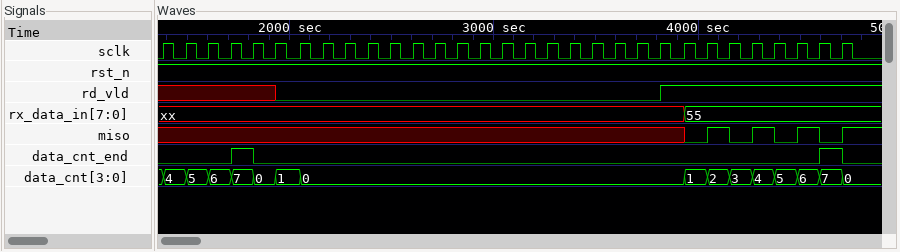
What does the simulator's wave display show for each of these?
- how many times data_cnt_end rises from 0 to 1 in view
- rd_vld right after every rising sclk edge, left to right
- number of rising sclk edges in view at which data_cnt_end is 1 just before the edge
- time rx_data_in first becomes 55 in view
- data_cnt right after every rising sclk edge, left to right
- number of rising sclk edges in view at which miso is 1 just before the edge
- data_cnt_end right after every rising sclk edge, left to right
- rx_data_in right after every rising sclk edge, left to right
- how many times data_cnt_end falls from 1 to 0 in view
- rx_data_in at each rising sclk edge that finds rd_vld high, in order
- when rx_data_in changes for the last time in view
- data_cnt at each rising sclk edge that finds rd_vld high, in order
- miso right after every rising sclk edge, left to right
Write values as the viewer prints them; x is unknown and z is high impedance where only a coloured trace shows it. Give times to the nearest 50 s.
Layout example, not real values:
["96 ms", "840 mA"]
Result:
["2", "x x x x x 0 0 0 0 0 0 0 0 0 0 0 0 0 0 0 0 0 1 1 1 1 1 1 1 1 1", "2", "3950 s", "4, 5, 6, 7, 0, 1, 0, 0, 0, 0, 0, 0, 0, 0, 0, 0, 0, 0, 0, 0, 0, 0, 0, 1, 2, 3, 4, 5, 6, 7, 0", "3", "0 0 0 1 0 0 0 0 0 0 0 0 0 0 0 0 0 0 0 0 0 0 0 0 0 0 0 0 0 1 0", "xx, xx, xx, xx, xx, xx, xx, xx, xx, xx, xx, xx, xx, xx, xx, xx, xx, xx, xx, xx, xx, xx, xx, 55, 55, 55, 55, 55, 55, 55, 55", "2", "xx, 55, 55, 55, 55, 55, 55, 55", "3950 s", "0, 1, 2, 3, 4, 5, 6, 7", "x x x x x x x x x x x x x x x x x x x x x x x 0 1 0 1 0 1 0 1"]
